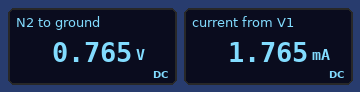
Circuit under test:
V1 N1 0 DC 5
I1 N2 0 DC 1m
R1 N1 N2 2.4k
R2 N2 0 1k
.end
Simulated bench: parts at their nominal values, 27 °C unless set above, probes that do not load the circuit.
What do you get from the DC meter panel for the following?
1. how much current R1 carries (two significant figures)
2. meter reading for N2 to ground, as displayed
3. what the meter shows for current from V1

1.8 mA
0.765 V
1.765 mA
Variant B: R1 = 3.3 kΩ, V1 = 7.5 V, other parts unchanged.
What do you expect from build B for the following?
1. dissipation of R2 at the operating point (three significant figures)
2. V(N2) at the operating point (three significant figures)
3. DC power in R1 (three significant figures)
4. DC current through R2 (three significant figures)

954 µW
977 mV
12.9 mW
977 µA
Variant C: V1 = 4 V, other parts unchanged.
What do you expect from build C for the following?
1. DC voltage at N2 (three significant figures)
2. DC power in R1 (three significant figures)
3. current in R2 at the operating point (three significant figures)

471 mV
5.19 mW
471 µA
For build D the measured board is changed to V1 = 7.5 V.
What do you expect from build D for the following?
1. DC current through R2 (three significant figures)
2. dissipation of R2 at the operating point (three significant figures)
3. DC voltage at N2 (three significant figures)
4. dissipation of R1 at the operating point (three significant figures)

1.50 mA
2.25 mW
1.50 V
15.0 mW
